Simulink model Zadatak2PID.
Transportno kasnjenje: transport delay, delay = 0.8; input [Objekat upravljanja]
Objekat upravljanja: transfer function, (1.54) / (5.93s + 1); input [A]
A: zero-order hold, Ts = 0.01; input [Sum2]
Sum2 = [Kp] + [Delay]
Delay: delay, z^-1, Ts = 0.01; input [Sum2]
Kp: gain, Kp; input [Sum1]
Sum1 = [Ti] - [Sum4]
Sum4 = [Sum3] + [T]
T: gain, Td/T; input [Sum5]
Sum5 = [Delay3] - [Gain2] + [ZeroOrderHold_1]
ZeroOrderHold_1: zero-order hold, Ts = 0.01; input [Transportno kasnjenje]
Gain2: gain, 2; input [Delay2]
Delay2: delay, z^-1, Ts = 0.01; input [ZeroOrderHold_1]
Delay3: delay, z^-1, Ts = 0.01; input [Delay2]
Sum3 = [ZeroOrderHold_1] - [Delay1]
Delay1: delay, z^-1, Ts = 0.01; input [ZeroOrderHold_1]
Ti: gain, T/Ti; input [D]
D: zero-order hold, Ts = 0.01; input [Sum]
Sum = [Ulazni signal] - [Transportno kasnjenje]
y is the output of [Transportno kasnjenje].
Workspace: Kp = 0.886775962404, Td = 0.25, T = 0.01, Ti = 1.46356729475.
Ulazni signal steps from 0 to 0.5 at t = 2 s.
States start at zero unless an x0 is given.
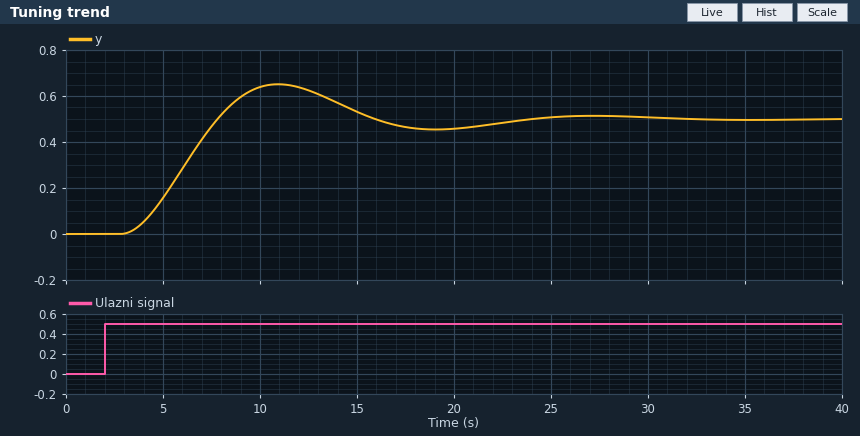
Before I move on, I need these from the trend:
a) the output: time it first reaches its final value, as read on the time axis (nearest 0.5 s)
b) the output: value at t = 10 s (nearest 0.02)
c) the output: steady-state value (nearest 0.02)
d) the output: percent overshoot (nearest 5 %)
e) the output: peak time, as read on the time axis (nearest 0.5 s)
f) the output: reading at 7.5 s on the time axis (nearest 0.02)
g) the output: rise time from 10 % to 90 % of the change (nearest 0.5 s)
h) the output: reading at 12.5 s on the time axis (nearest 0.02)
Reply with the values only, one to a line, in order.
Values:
8.0 s
0.64
0.50
30 %
11.0 s
0.46
3.5 s
0.62
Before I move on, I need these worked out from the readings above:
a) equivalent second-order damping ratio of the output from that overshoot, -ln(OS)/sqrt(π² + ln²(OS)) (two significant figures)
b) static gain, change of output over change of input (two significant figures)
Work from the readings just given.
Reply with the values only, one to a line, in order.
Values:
0.36
1.0
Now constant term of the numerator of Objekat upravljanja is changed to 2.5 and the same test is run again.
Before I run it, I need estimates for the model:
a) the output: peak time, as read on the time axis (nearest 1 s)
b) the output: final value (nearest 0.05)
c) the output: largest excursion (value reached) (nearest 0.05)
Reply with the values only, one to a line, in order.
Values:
9 s
0.50
0.65
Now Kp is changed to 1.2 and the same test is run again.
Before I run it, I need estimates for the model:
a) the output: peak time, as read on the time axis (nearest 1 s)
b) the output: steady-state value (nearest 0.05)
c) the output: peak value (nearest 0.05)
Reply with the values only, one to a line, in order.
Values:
10 s
0.50
0.65
